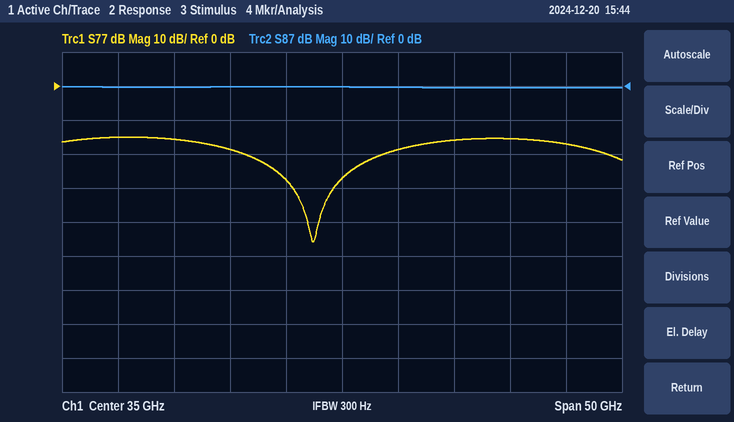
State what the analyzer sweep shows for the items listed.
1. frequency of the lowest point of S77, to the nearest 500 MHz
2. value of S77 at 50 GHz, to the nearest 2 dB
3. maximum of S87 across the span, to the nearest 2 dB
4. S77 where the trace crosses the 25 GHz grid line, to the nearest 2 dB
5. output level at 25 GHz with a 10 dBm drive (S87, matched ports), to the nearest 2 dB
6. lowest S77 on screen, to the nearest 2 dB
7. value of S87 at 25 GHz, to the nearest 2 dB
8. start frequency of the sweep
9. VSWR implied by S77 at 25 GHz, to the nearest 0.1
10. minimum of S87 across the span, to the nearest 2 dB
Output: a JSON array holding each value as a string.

["32.5 GHz", "-16 dB", "0 dB", "-18 dB", "10 dBm", "-46 dB", "0 dB", "10 GHz", "1.3", "0 dB"]
